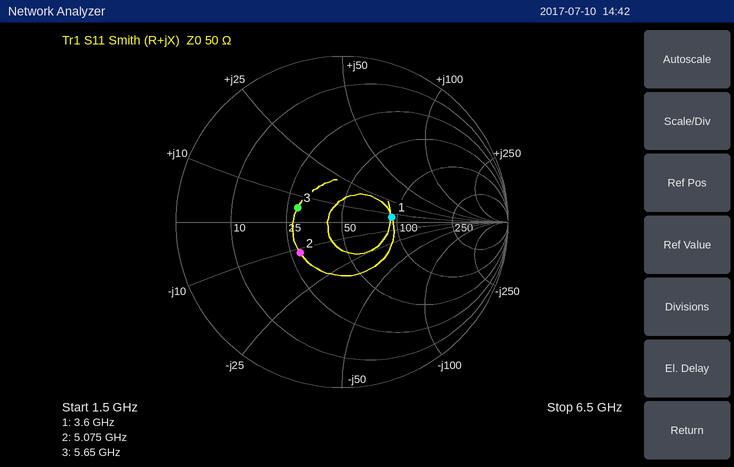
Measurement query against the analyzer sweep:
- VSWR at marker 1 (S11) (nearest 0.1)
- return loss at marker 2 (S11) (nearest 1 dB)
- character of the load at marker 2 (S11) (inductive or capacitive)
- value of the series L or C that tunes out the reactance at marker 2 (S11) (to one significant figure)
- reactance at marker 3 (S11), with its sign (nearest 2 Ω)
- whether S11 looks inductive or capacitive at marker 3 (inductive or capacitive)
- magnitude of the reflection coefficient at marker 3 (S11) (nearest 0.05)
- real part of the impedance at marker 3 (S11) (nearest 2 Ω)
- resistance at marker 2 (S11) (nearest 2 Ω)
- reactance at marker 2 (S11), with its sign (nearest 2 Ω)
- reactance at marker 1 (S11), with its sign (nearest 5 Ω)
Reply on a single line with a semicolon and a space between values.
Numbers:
1.9; 10 dB; capacitive; 400 pH; +6 Ω; inductive; 0.30; 28 Ω; 28 Ω; -12 Ω; +5 Ω
